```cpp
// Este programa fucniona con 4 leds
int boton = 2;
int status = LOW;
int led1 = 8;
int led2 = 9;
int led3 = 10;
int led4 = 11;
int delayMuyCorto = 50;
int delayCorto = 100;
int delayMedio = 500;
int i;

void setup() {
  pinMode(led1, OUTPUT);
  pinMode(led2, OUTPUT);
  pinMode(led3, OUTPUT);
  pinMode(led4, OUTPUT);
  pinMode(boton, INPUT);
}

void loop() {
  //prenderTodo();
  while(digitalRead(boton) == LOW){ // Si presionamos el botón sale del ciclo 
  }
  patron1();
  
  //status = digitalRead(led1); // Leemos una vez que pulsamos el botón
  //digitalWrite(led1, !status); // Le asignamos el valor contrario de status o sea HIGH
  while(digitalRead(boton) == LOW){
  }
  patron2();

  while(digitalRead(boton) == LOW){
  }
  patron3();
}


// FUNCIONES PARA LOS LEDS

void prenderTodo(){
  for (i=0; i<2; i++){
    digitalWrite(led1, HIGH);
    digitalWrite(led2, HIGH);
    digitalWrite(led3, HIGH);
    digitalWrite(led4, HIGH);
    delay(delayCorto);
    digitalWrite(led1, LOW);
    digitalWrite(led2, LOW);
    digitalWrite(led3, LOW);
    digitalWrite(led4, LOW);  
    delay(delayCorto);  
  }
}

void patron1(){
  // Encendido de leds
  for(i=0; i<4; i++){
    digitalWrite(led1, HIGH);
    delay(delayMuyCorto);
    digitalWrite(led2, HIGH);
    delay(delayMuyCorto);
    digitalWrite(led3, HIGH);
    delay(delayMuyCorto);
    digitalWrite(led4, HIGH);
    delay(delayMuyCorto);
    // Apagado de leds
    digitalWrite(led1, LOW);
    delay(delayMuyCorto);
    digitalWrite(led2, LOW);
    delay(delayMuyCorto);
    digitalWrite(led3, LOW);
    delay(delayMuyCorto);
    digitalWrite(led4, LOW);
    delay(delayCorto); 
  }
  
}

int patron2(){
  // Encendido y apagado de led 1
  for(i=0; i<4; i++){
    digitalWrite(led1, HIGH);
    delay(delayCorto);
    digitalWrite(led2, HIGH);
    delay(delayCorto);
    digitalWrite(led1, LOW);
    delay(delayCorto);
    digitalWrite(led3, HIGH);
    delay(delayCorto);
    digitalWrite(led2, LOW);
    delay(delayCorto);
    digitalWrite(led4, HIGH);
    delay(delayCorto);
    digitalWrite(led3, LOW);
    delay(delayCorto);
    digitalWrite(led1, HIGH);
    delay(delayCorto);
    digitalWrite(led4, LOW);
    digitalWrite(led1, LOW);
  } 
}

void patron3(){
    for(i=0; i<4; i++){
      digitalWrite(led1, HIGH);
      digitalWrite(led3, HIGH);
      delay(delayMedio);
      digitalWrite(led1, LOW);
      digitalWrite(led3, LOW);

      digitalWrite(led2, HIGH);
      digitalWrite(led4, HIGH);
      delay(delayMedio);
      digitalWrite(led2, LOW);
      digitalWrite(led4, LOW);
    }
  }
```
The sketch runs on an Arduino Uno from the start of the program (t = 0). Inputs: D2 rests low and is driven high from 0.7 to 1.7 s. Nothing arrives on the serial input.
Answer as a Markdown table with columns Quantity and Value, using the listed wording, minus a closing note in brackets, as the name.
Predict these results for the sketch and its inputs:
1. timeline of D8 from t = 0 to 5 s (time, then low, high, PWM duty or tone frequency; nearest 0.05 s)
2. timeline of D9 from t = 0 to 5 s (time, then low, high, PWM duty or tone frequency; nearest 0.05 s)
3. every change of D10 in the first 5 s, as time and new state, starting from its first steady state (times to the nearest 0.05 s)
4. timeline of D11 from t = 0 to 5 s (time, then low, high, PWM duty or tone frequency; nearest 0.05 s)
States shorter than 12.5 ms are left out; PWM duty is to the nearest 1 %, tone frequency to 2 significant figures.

| Quantity | Value |
|---|---|
| timeline of D8 from t = 0 to 5 s | 0 s low; 0.7 s high; 0.9 s low; 1.15 s high; 1.35 s low; 1.6 s high; 1.8 s low; 2.05 s high; 2.25 s low |
| timeline of D9 from t = 0 to 5 s | 0 s low; 0.75 s high; 0.95 s low; 1.2 s high; 1.4 s low; 1.65 s high; 1.85 s low; 2.1 s high; 2.3 s low |
| every change of D10 in the first 5 s, as time and new state, starting from its first steady state | 0 s low; 0.8 s high; 1 s low; 1.25 s high; 1.45 s low; 1.7 s high; 1.9 s low; 2.15 s high; 2.35 s low |
| timeline of D11 from t = 0 to 5 s | 0 s low; 0.85 s high; 1.05 s low; 1.3 s high; 1.5 s low; 1.75 s high; 1.95 s low; 2.2 s high; 2.4 s low |
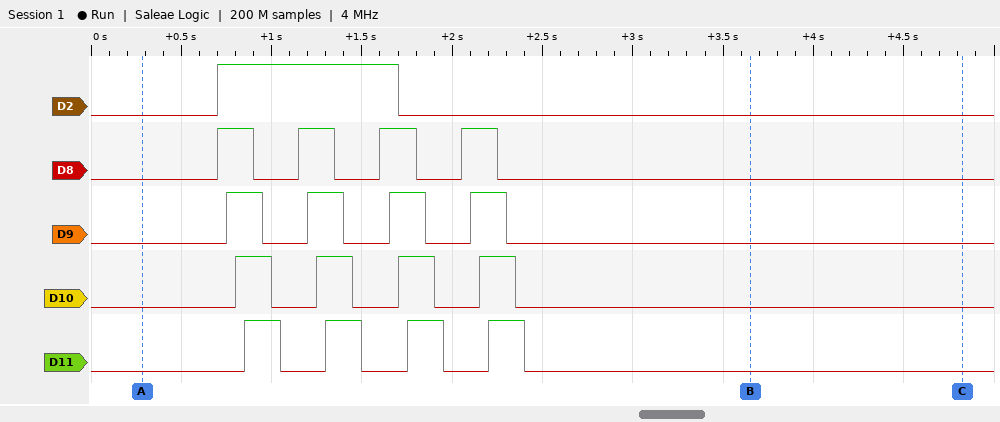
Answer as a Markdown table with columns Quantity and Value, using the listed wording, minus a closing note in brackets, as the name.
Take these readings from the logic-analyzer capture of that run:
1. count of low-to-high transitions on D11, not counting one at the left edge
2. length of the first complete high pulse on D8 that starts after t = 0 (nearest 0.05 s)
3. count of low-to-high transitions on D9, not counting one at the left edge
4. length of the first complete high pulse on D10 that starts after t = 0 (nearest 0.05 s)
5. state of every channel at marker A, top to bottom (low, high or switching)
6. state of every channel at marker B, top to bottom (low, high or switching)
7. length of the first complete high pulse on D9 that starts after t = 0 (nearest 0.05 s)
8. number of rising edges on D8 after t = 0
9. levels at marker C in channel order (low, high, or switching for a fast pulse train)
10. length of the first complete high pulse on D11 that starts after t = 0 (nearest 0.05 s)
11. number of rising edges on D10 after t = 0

| Quantity | Value |
|---|---|
| count of low-to-high transitions on D11, not counting one at the left edge | 4 |
| length of the first complete high pulse on D8 that starts after t = 0 | 0.20 s |
| count of low-to-high transitions on D9, not counting one at the left edge | 4 |
| length of the first complete high pulse on D10 that starts after t = 0 | 0.20 s |
| state of every channel at marker A, top to bottom | D2 low, D8 low, D9 low, D10 low, D11 low |
| state of every channel at marker B, top to bottom | D2 low, D8 low, D9 low, D10 low, D11 low |
| length of the first complete high pulse on D9 that starts after t = 0 | 0.20 s |
| number of rising edges on D8 after t = 0 | 4 |
| levels at marker C in channel order | D2 low, D8 low, D9 low, D10 low, D11 low |
| length of the first complete high pulse on D11 that starts after t = 0 | 0.20 s |
| number of rising edges on D10 after t = 0 | 4 |
